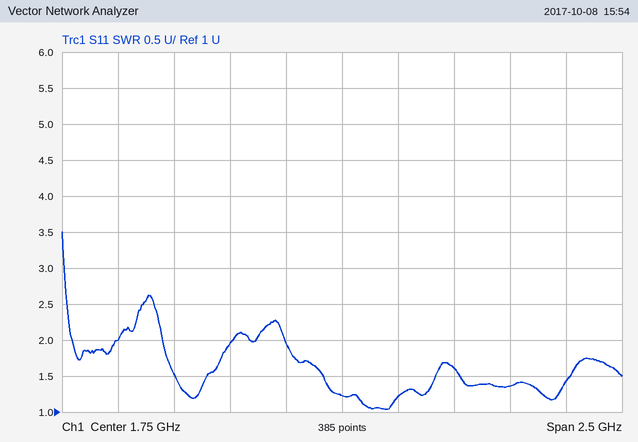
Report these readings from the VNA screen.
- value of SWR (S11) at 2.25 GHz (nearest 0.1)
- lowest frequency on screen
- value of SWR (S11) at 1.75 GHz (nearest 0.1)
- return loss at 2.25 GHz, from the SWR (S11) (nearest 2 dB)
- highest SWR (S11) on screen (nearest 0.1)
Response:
1.6
500 MHz
1.2
12 dB
3.5
